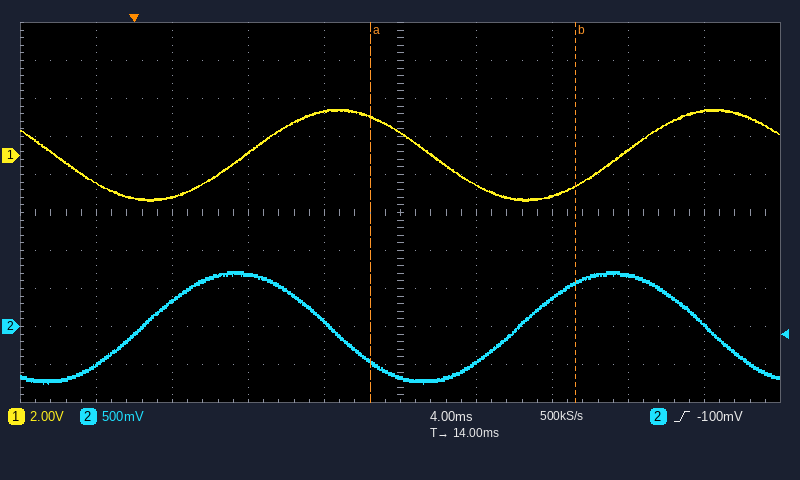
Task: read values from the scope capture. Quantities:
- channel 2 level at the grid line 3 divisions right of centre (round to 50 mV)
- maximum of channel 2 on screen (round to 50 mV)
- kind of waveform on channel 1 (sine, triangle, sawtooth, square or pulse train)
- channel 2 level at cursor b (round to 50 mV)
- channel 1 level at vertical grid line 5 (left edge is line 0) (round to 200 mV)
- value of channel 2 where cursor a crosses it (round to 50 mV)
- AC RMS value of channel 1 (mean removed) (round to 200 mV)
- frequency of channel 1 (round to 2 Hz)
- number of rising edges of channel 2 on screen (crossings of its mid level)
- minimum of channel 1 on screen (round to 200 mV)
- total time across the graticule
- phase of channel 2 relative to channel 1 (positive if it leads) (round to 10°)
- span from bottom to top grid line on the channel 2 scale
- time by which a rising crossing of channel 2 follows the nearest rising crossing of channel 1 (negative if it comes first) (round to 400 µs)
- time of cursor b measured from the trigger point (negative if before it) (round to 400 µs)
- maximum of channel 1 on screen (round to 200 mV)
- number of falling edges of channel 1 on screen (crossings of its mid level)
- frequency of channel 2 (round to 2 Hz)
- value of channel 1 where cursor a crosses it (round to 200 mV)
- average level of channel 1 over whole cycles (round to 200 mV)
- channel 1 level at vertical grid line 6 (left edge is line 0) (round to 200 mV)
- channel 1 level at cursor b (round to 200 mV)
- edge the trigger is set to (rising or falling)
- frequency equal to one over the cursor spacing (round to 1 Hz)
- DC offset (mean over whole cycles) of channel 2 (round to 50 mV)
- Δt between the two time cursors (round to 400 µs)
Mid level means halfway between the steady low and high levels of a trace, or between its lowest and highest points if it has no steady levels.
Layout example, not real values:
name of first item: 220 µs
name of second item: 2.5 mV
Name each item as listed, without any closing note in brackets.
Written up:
channel 2 level at the grid line 3 divisions right of centre: 650 mV
maximum of channel 2 on screen: 700 mV
kind of waveform on channel 1: sine
channel 2 level at cursor b: 550 mV
channel 1 level at vertical grid line 5 (left edge is line 0): 1.2 V
value of channel 2 where cursor a crosses it: -450 mV
AC RMS value of channel 1 (mean removed): 1.6 V
frequency of channel 1: 50 Hz
number of rising edges of channel 2 on screen: 2
minimum of channel 1 on screen: -2.4 V
total time across the graticule: 40 ms
phase of channel 2 relative to channel 1 (positive if it leads): +100°
span from bottom to top grid line on the channel 2 scale: 5 V
time by which a rising crossing of channel 2 follows the nearest rising crossing of channel 1 (negative if it comes first): -5.6 ms
time of cursor b measured from the trigger point (negative if before it): +23.2 ms
maximum of channel 1 on screen: 2.4 V
number of falling edges of channel 1 on screen: 2
frequency of channel 2: 50 Hz
value of channel 1 where cursor a crosses it: 2.0 V
average level of channel 1 over whole cycles: 0.0 V
channel 1 level at vertical grid line 6 (left edge is line 0): -1.6 V
channel 1 level at cursor b: -1.6 V
edge the trigger is set to: rising
frequency equal to one over the cursor spacing: 93 Hz
DC offset (mean over whole cycles) of channel 2: 0 mV
Δt between the two time cursors: 10.8 ms
